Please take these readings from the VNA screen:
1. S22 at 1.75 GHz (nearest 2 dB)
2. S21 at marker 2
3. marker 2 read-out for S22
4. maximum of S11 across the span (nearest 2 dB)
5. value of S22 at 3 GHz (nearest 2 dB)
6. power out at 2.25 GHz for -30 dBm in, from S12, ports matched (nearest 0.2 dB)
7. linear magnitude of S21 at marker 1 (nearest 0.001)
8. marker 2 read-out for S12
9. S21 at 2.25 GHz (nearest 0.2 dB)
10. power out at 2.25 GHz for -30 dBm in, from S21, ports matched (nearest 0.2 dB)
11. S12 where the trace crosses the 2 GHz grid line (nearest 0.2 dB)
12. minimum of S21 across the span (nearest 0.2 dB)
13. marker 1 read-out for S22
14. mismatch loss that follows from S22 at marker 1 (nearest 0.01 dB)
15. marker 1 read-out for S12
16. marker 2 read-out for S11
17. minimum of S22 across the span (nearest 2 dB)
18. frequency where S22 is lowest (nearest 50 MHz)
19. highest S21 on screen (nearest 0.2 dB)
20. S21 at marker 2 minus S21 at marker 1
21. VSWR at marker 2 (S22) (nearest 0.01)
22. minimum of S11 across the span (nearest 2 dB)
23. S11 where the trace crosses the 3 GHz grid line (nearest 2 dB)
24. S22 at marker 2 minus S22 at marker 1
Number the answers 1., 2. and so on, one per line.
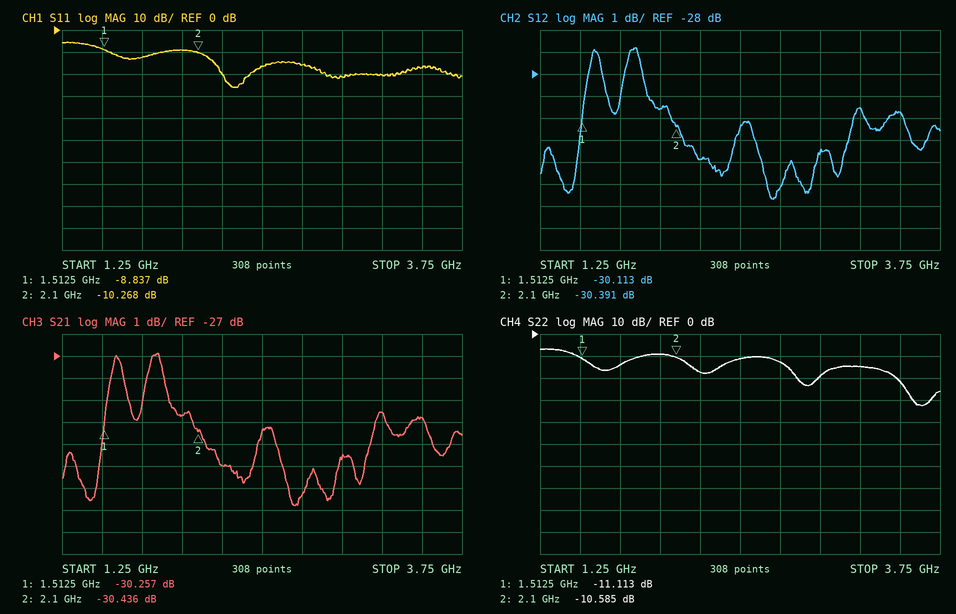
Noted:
1. -14 dB
2. -30.436 dB
3. -10.585 dB
4. -6 dB
5. -20 dB
6. -61.8 dBm
7. 0.031
8. -30.391 dB
9. -32.0 dB
10. -62.0 dBm
11. -29.6 dB
12. -33.8 dB
13. -11.113 dB
14. 0.35 dB
15. -30.113 dB
16. -10.268 dB
17. -32 dB
18. 3.65 GHz
19. -26.8 dB
20. -0.179 dB
21. 1.84
22. -26 dB
23. -22 dB
24. 0.528 dB
